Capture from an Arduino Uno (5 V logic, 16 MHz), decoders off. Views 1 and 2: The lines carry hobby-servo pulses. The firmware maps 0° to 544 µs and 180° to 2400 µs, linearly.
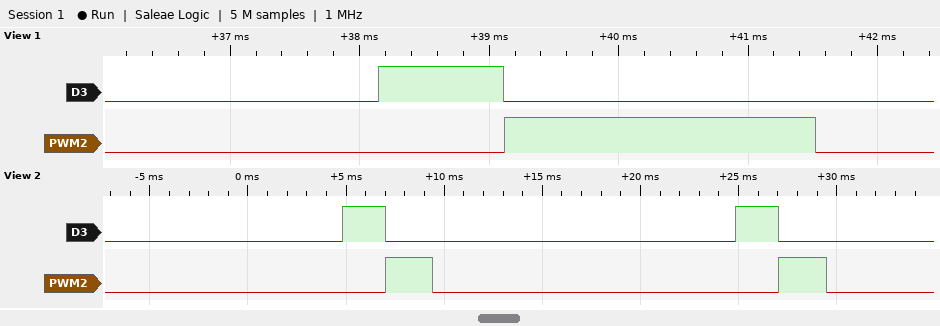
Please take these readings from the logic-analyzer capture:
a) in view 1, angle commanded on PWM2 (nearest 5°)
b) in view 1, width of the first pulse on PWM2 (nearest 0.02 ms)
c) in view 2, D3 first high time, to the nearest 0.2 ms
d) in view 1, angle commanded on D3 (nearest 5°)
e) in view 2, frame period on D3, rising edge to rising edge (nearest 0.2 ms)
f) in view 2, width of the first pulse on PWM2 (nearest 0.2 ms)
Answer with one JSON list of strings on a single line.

["180°", "2.40 ms", "2.2 ms", "40°", "20.0 ms", "2.4 ms"]
